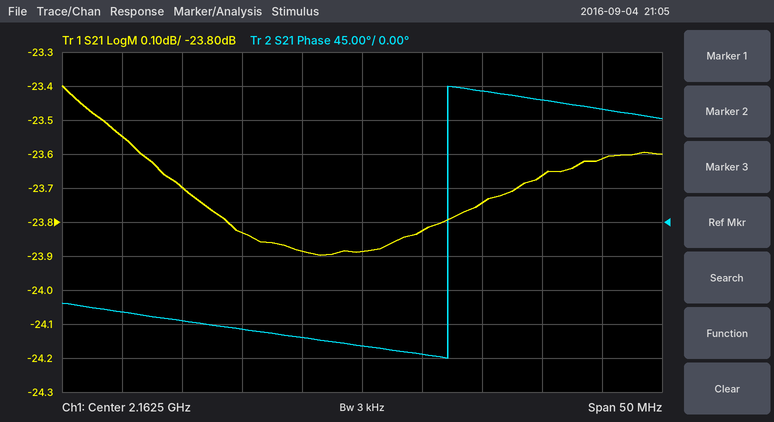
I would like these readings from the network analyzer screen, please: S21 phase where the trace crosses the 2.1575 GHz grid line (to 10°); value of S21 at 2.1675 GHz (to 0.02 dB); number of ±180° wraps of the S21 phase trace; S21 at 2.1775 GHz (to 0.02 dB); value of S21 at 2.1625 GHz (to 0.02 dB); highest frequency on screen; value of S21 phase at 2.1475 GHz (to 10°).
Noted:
-150°
-23.82 dB
1
-23.66 dB
-23.88 dB
2.1875 GHz
-130°
